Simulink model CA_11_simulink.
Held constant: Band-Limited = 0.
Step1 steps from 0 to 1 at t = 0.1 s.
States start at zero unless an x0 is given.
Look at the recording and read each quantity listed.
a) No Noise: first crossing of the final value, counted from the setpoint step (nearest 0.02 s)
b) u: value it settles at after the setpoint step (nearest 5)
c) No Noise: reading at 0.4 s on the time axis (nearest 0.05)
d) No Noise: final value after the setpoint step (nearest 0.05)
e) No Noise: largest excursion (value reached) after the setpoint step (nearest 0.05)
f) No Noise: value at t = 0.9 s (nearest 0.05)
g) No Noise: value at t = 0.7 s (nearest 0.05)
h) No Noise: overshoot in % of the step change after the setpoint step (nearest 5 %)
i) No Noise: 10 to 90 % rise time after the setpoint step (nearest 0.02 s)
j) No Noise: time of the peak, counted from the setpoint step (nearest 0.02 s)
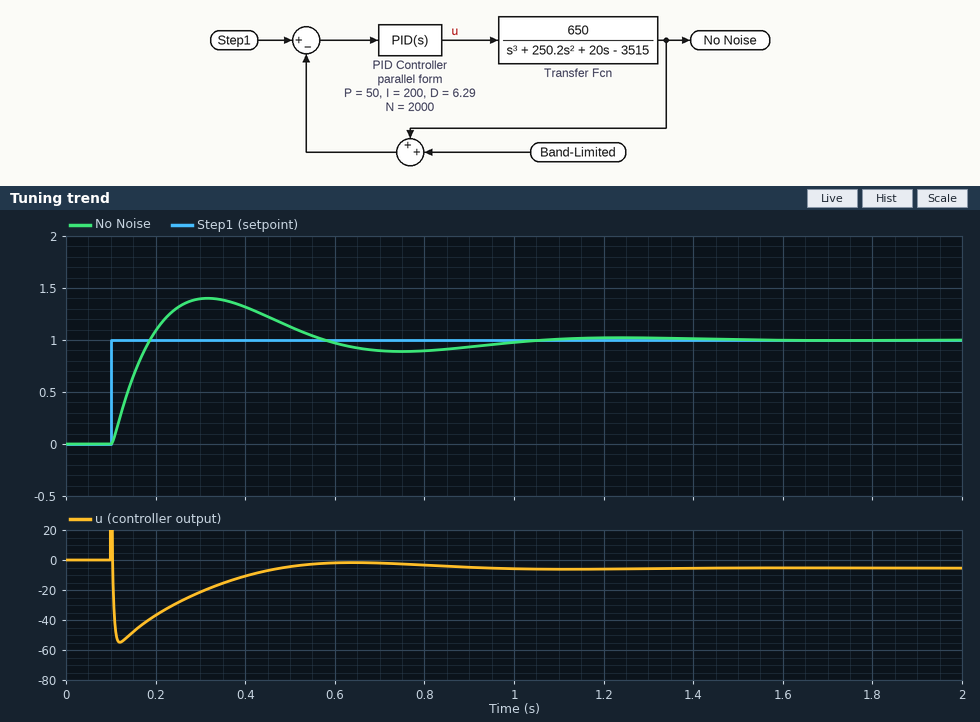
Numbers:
0.08 s
-5
1.30
1.00
1.40
0.95
0.90
40 %
0.06 s
0.22 s
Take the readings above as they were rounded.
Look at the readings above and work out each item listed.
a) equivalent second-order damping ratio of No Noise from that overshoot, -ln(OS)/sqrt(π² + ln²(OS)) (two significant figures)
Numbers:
0.28
